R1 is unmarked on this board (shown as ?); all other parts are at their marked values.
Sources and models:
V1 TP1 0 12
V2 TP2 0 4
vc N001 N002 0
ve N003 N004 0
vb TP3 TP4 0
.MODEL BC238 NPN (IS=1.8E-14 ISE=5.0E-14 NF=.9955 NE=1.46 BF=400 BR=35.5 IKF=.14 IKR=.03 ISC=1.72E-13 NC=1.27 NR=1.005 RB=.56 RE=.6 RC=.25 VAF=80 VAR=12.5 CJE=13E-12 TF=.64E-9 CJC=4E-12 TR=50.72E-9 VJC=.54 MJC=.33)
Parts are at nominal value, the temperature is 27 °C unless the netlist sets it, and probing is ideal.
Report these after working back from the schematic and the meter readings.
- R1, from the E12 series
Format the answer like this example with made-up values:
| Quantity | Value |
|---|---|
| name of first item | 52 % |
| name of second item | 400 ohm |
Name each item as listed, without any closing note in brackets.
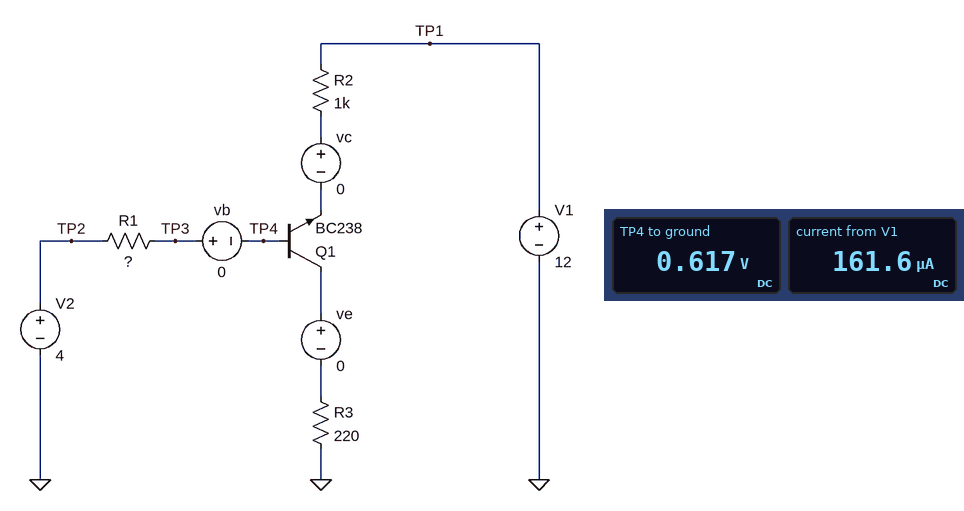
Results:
| Quantity | Value |
|---|---|
| R1, from the E12 series | 330 kΩ |
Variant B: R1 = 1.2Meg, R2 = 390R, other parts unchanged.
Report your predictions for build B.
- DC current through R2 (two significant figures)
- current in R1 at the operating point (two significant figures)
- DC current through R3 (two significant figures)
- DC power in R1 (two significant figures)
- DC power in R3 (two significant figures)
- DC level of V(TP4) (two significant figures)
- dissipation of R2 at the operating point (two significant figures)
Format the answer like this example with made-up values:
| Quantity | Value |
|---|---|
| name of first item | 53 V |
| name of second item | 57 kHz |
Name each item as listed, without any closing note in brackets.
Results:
| Quantity | Value |
|---|---|
| DC current through R2 | 36 µA |
| current in R1 at the operating point | 2.9 µA |
| DC current through R3 | 39 µA |
| DC power in R1 | 9.9 µW |
| DC power in R3 | 330 nW |
| DC level of V(TP4) | 550 mV |
| dissipation of R2 at the operating point | 500 nW |
